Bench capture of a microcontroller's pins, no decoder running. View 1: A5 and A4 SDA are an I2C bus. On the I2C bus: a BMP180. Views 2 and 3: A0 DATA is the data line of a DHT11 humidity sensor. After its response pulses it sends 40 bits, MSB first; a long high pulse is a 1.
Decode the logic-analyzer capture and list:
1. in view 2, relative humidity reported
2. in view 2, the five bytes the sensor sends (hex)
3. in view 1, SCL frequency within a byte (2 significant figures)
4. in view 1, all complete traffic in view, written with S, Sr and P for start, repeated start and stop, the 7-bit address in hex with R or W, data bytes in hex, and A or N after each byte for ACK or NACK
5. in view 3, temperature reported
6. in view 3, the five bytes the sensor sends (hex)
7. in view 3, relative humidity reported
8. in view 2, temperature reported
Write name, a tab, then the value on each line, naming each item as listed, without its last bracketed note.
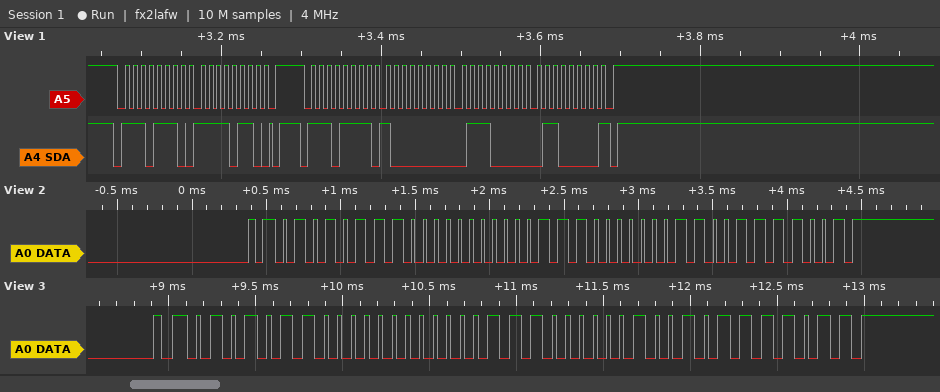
in view 2, relative humidity reported	87 %
in view 2, the five bytes the sensor sends	57 00 1C 06 79
in view 1, SCL frequency within a byte	100 kHz
in view 1, all complete traffic in view, written with S, Sr and P for start, repeated start and stop, the 7-bit address in hex with R or W, data bytes in hex, and A or N after each byte for ACK or NACK	S 77W A F6 A P S 77R A 80 A 70 A 60 N P
in view 3, temperature reported	28.9 °C
in view 3, the five bytes the sensor sends	56 00 1C 09 7B
in view 3, relative humidity reported	86 %
in view 2, temperature reported	28.6 °C
